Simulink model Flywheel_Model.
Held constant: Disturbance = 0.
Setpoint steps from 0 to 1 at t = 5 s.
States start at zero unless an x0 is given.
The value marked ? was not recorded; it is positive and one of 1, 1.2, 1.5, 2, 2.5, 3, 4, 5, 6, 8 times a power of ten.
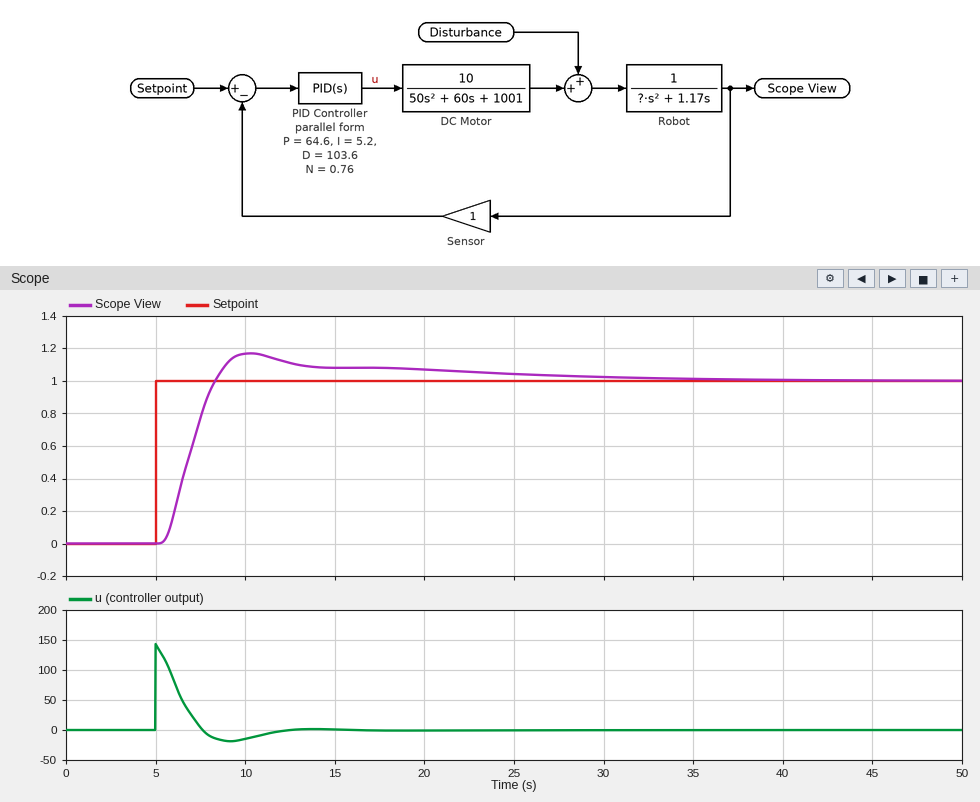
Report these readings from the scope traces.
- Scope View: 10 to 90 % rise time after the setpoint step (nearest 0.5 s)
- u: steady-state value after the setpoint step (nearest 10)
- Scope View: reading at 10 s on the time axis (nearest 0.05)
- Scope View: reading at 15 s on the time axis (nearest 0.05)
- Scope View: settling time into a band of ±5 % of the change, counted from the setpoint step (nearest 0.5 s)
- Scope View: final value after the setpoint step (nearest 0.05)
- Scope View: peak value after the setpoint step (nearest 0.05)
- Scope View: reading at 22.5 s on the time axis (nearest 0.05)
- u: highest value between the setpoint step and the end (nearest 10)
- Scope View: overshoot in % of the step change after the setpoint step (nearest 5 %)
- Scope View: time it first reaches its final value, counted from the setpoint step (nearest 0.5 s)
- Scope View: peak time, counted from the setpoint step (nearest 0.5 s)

2.0 s
0
1.15
1.10
18.5 s
1.00
1.15
1.05
140
15 %
3.5 s
5.5 s
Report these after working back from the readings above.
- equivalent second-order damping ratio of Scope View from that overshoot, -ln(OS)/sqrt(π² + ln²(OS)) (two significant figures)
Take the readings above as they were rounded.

0.52
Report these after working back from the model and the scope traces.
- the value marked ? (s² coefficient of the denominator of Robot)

2.5
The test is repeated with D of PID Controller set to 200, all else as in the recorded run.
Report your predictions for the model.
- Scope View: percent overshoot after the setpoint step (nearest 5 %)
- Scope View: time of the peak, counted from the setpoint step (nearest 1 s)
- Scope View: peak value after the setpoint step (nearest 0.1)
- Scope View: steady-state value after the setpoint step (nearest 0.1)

10 %
4 s
1.1
1.0
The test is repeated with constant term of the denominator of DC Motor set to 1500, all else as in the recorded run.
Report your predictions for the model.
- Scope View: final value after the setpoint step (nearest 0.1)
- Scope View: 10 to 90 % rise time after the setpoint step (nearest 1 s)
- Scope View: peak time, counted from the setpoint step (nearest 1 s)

1.0
3 s
9 s
